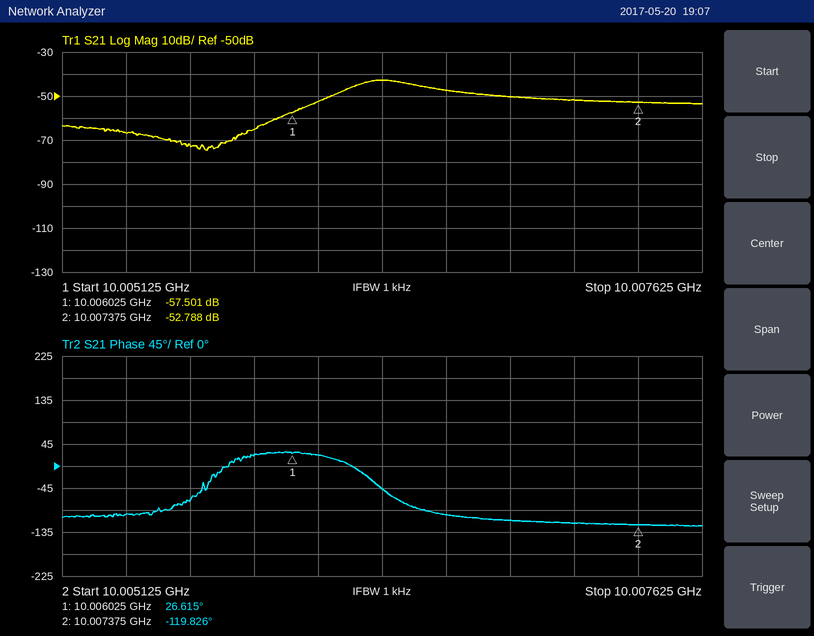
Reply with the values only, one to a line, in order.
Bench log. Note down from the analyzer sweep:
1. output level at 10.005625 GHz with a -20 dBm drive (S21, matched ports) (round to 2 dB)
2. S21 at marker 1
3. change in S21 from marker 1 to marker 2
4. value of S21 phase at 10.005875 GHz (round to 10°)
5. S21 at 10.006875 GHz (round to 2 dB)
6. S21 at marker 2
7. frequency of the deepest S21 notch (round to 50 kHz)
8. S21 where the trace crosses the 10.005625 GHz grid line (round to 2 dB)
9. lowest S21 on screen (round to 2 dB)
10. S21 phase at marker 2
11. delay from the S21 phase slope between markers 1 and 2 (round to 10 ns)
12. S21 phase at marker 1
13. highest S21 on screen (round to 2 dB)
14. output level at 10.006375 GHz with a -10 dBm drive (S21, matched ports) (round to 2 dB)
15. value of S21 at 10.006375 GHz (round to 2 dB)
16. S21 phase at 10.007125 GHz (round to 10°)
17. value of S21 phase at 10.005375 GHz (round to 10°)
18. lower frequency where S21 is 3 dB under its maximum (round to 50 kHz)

-92 dBm
-57.501 dB
4.713 dB
20°
-50 dB
-52.788 dB
10.00570 GHz
-72 dB
-74 dB
-119.826°
300 ns
26.615°
-42 dB
-52 dBm
-42 dB
-120°
-100°
10.00625 GHz
